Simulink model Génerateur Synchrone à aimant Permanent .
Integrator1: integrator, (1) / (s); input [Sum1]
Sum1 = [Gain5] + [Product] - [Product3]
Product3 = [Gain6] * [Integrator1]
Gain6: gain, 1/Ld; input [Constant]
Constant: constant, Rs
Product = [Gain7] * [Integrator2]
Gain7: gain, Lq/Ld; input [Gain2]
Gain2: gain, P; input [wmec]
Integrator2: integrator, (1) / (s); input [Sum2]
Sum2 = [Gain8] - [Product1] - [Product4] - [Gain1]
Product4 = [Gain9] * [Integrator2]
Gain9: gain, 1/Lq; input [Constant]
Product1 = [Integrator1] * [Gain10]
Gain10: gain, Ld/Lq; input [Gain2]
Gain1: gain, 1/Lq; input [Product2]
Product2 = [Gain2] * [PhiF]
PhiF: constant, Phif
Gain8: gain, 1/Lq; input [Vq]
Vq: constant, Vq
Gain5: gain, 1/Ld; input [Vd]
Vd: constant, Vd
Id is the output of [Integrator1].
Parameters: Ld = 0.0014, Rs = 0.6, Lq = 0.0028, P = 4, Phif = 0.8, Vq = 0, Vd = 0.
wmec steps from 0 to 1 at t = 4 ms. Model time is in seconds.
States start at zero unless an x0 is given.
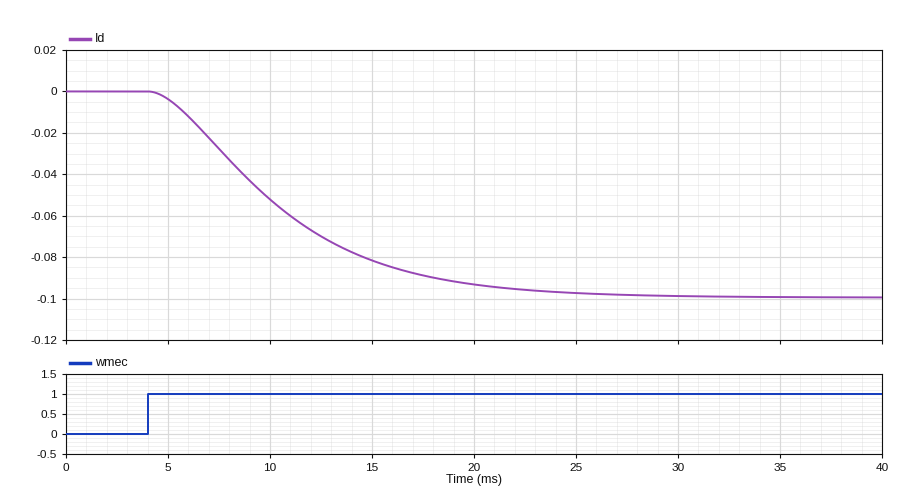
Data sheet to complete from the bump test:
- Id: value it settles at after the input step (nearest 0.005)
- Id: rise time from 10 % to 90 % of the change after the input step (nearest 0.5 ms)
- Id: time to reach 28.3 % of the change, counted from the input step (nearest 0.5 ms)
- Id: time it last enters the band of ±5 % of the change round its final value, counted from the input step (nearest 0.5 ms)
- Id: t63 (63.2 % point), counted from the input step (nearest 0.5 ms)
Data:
-0.100
12.0 ms
3.5 ms
17.0 ms
7.5 ms
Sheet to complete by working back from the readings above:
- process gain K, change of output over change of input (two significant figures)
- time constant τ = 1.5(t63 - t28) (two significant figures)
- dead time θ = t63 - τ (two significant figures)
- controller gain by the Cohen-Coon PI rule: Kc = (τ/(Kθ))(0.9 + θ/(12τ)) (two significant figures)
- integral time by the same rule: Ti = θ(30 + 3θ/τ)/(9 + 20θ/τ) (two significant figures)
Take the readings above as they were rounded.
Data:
-0.10
6.0 ms
1.5 ms
-37
3.3 ms
